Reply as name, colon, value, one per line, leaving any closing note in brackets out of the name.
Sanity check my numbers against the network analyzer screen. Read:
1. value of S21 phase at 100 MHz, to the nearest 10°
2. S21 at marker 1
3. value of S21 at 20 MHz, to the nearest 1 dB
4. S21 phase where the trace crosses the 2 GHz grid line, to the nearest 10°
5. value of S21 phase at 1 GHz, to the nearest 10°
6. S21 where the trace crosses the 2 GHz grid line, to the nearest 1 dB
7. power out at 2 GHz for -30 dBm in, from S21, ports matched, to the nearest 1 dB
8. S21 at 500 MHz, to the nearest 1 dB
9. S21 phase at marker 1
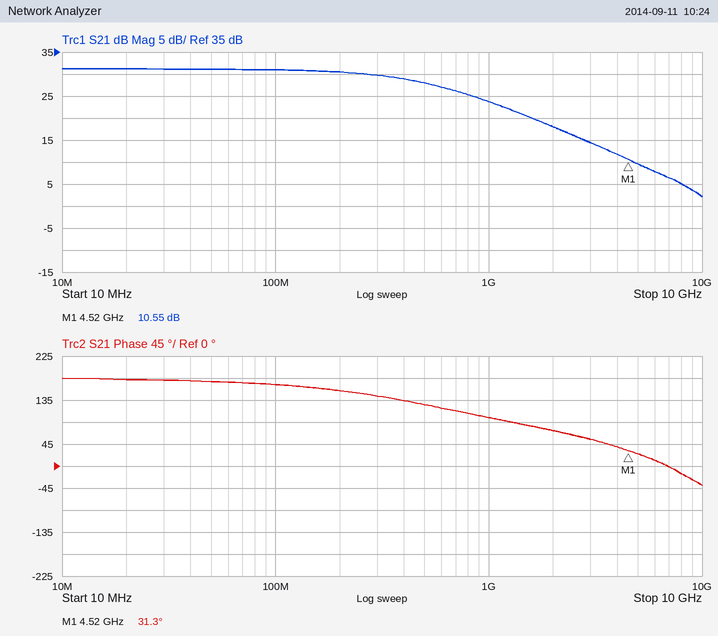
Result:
value of S21 phase at 100 MHz, to the nearest 10°: 170°
S21 at marker 1: 10.55 dB
value of S21 at 20 MHz, to the nearest 1 dB: 31 dB
S21 phase where the trace crosses the 2 GHz grid line, to the nearest 10°: 70°
value of S21 phase at 1 GHz, to the nearest 10°: 100°
S21 where the trace crosses the 2 GHz grid line, to the nearest 1 dB: 18 dB
power out at 2 GHz for -30 dBm in, from S21, ports matched, to the nearest 1 dB: -12 dBm
S21 at 500 MHz, to the nearest 1 dB: 28 dB
S21 phase at marker 1: 31.3°
